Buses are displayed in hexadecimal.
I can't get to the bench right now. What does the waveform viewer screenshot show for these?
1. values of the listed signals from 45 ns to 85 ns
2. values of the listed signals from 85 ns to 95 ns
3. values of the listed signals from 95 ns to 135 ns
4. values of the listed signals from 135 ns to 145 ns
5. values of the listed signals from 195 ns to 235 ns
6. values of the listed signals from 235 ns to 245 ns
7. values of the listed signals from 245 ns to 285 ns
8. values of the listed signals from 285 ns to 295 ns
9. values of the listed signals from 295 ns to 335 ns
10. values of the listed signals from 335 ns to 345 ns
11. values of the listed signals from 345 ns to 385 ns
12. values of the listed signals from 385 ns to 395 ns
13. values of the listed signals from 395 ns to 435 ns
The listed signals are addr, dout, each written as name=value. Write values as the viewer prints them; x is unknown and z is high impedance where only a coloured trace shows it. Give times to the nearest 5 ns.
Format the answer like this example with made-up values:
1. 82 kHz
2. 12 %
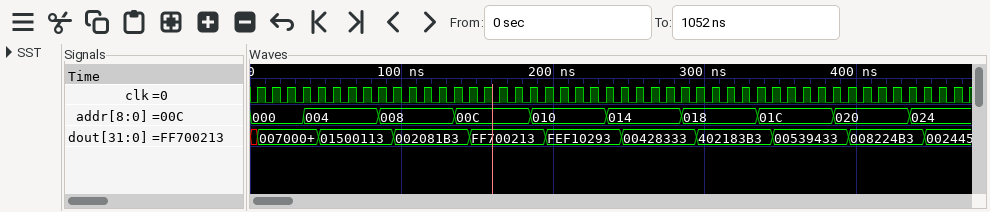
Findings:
1. addr=004, dout=01500113
2. addr=008, dout=01500113
3. addr=008, dout=002081B3
4. addr=00C, dout=002081B3
5. addr=010, dout=FEF10293
6. addr=014, dout=FEF10293
7. addr=014, dout=00428333
8. addr=018, dout=00428333
9. addr=018, dout=402183B3
10. addr=01C, dout=402183B3
11. addr=01C, dout=00539433
12. addr=020, dout=00539433
13. addr=020, dout=008224B3
